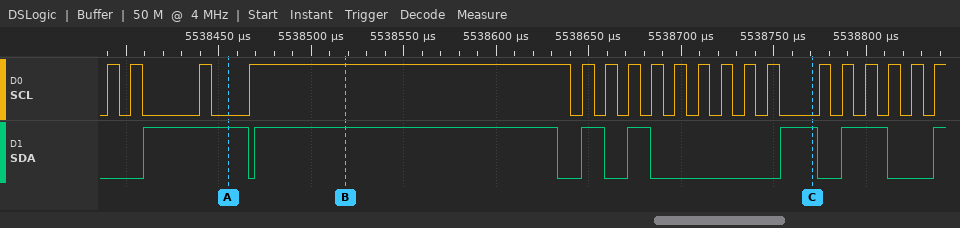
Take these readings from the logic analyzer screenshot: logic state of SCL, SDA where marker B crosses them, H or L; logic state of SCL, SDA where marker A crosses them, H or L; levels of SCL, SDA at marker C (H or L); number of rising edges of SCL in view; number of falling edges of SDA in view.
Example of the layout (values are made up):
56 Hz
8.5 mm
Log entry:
SCL=H, SDA=H
SCL=L, SDA=H
SCL=L, SDA=H
19
6
